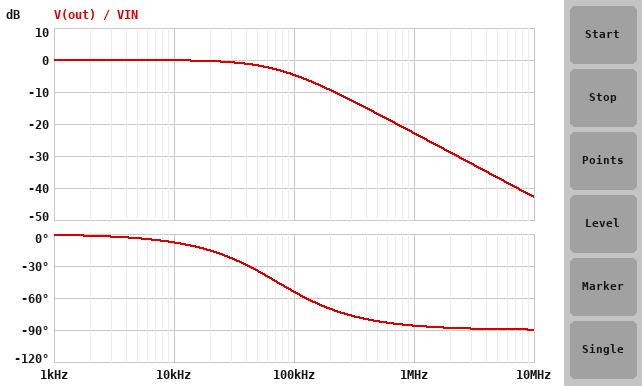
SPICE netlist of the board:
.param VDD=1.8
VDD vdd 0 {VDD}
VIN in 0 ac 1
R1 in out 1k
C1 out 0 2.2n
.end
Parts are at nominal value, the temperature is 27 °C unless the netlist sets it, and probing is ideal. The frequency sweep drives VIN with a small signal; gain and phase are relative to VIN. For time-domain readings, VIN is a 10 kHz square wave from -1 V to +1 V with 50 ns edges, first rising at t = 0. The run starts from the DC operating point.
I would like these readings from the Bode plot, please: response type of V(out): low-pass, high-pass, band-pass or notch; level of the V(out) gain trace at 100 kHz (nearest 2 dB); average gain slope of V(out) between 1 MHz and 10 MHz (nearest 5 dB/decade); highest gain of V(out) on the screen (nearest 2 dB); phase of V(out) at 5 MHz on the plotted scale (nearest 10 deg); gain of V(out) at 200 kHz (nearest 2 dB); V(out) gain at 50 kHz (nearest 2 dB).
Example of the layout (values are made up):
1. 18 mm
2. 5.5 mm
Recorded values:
1. low-pass
2. -4 dB
3. -20 dB/decade
4. 0 dB
5. -90 deg
6. -10 dB
7. -2 dB
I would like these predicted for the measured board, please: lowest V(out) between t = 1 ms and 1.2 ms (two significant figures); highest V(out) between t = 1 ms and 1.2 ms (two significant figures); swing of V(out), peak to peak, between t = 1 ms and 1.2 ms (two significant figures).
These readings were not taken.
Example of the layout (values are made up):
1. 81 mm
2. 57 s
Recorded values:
1. -1.0 V
2. 1.0 V
3. 2.0 V
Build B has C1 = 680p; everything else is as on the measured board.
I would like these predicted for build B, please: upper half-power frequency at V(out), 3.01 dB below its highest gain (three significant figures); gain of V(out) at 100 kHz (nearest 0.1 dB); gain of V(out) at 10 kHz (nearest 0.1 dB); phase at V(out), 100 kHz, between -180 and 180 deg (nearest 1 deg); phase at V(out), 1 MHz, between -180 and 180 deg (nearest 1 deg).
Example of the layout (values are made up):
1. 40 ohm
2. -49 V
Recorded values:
1. 234 kHz
2. -0.7 dB
3. 0 dB
4. -23 deg
5. -77 deg
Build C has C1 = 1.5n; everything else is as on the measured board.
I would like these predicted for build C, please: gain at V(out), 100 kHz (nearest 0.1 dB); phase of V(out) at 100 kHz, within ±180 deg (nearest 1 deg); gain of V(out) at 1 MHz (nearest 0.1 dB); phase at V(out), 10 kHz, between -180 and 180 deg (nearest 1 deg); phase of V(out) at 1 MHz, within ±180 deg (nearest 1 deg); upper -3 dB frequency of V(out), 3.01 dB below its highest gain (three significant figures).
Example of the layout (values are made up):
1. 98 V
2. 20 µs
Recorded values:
1. -2.8 dB
2. -43 deg
3. -19.5 dB
4. -5 deg
5. -84 deg
6. 106 kHz
